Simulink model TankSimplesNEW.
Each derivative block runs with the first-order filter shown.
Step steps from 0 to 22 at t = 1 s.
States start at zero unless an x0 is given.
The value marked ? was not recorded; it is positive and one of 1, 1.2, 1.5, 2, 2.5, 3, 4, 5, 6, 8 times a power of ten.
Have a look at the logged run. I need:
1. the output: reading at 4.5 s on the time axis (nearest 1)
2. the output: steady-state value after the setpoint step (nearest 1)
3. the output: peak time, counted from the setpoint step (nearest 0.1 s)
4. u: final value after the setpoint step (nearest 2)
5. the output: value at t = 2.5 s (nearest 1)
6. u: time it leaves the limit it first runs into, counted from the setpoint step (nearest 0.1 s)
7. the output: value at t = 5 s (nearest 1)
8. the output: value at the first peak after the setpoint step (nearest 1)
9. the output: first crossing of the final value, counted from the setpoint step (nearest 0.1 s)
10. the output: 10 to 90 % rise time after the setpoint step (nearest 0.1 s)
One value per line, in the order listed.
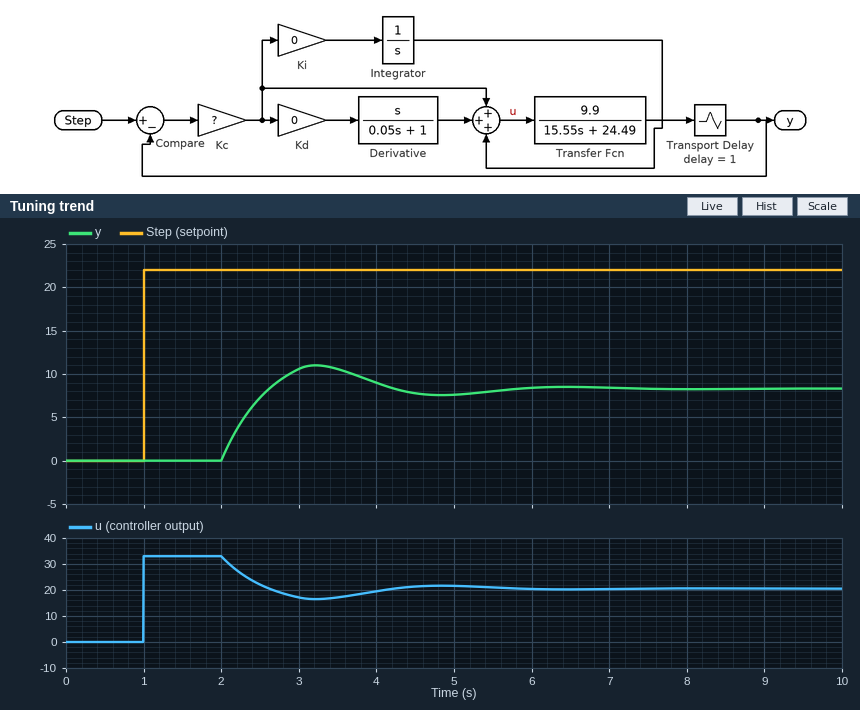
8
8
2.2 s
20
7
1.0 s
8
11
1.6 s
0.5 s
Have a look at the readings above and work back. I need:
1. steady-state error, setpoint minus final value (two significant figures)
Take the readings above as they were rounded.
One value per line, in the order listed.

14
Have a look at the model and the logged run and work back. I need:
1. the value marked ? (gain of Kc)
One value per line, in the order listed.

1.5
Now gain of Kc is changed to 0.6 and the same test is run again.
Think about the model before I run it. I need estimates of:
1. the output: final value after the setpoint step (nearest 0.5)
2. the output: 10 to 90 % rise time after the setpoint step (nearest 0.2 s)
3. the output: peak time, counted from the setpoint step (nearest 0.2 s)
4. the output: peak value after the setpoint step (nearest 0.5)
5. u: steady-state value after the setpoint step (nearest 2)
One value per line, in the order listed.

4.5
0.8 s
2.6 s
4.5
10
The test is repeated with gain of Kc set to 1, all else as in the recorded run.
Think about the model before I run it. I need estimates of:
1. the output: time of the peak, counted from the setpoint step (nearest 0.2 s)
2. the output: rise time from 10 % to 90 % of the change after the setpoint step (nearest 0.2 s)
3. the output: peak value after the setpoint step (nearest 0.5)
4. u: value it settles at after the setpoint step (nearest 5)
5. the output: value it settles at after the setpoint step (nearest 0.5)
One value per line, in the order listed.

2.4 s
0.6 s
7.5
15
6.5
